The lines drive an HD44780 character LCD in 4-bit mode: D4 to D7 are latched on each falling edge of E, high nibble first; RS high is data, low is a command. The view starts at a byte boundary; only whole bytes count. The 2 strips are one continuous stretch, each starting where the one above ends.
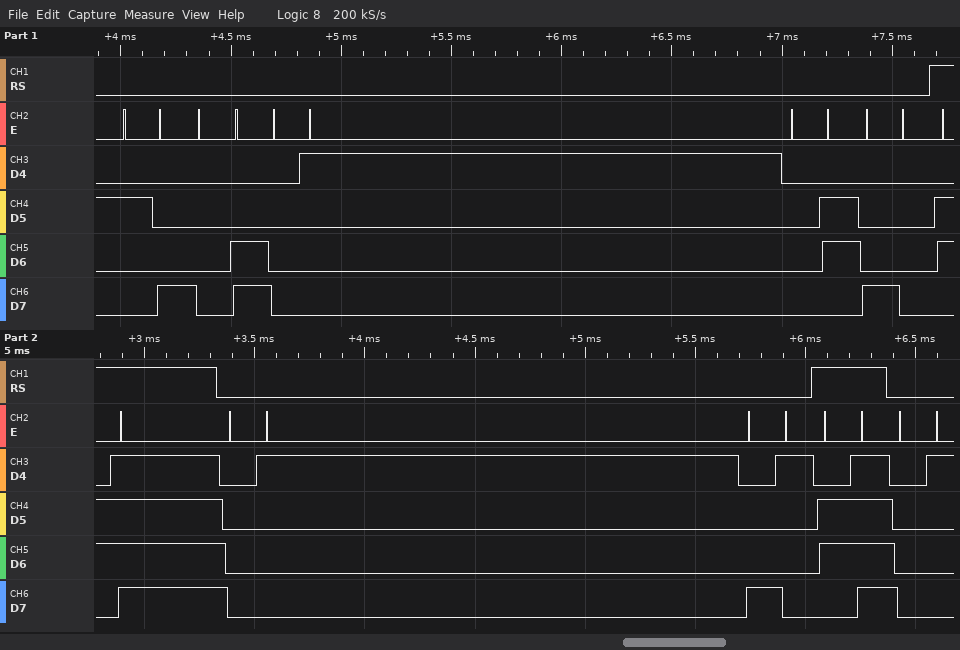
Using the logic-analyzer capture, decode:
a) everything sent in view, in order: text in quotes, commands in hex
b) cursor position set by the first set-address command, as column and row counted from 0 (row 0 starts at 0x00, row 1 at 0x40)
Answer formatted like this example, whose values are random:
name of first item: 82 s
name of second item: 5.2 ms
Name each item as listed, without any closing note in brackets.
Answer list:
everything sent in view, in order: text in quotes, commands in hex: 0x28 0x0C 0x01 0x06 0x80 "o" 0x01 0x81 "o" 0x01
cursor position set by the first set-address command, as column and row counted from 0: column 0, row 0
